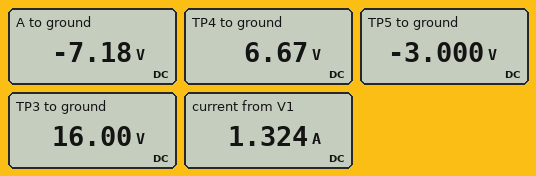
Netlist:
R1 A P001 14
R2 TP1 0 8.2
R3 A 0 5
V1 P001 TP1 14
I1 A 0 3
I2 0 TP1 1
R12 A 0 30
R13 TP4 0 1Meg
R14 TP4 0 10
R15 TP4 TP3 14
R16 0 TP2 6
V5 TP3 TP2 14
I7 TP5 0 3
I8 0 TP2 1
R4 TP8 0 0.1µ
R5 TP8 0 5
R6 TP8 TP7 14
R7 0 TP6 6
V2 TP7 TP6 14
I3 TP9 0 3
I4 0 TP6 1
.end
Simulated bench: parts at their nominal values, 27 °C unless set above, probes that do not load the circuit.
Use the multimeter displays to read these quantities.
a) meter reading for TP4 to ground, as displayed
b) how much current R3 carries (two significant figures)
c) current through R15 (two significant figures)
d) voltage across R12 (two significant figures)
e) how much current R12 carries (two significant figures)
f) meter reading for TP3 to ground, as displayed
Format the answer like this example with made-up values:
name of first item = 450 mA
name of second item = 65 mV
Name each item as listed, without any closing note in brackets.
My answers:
meter reading for TP4 to ground, as displayed = 6.67 V
how much current R3 carries = 1.4 A
current through R15 = 670 mA
voltage across R12 = 7.2 V
how much current R12 carries = 240 mA
meter reading for TP3 to ground, as displayed = 16.00 V
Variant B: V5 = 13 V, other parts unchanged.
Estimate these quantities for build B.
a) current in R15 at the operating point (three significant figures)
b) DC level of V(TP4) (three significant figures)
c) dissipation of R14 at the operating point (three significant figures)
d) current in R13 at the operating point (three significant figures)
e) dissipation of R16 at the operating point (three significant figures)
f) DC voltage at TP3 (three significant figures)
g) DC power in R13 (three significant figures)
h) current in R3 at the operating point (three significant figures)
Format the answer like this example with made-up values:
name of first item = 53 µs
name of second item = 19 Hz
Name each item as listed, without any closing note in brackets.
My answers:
current in R15 at the operating point = 633 mA
DC level of V(TP4) = 6.33 V
dissipation of R14 at the operating point = 4.01 W
current in R13 at the operating point = 6.33 µA
dissipation of R16 at the operating point = 807 mW
DC voltage at TP3 = 15.2 V
DC power in R13 = 40.1 µW
current in R3 at the operating point = 1.44 A
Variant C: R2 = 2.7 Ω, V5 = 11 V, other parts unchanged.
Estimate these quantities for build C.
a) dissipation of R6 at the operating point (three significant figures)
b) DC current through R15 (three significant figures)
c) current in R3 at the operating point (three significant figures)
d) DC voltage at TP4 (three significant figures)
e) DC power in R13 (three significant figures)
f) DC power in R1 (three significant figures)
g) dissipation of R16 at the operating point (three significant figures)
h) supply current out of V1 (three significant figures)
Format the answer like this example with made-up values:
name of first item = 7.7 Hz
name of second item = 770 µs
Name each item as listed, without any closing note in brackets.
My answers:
dissipation of R6 at the operating point = 14.0 W
DC current through R15 = 567 mA
current in R3 at the operating point = 1.36 A
DC voltage at TP4 = 5.67 V
DC power in R13 = 32.1 µW
DC power in R1 = 27.8 W
dissipation of R16 at the operating point = 1.13 W
supply current out of V1 = 1.41 A
